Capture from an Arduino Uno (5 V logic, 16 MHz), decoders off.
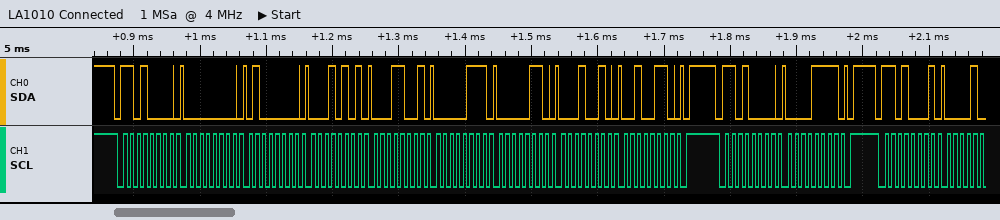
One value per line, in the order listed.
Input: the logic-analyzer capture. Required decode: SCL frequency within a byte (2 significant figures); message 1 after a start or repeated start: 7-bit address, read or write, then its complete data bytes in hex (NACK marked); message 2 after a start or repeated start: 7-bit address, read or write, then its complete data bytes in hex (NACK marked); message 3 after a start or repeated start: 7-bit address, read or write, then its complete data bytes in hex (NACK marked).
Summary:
100 kHz
0x68 write: 00 40 15 19 07 06 12 26
0x68 write: 0F
0x68 read
